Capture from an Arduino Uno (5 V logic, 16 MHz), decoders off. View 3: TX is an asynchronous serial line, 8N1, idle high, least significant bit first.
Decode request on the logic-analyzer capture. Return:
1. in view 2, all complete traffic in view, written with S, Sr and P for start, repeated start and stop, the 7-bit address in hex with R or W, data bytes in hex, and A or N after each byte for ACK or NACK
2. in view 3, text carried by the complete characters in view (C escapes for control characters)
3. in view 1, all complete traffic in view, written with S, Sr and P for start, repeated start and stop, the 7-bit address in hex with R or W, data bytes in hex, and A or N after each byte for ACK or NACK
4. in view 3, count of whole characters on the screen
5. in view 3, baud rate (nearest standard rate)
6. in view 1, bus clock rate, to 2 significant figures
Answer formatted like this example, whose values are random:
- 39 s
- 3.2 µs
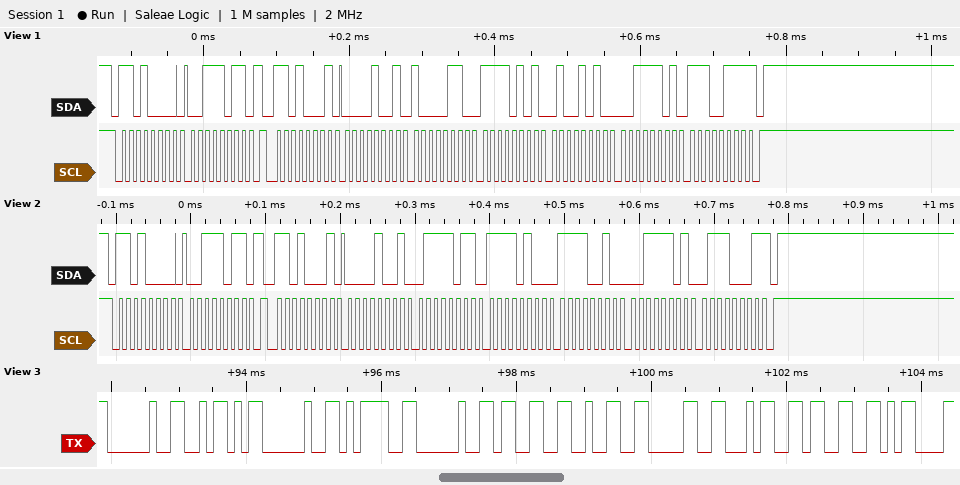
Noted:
- S 68W A 3B A Sr 68R A 09 A 7B A F4 A F2 A 3D A 71 N P
- " Z = 32043\r"
- S 68W A 3B A Sr 68R A 09 A 86 A F5 A 4A A 3D A E7 N P
- 11
- 9600 baud
- 100 kHz
